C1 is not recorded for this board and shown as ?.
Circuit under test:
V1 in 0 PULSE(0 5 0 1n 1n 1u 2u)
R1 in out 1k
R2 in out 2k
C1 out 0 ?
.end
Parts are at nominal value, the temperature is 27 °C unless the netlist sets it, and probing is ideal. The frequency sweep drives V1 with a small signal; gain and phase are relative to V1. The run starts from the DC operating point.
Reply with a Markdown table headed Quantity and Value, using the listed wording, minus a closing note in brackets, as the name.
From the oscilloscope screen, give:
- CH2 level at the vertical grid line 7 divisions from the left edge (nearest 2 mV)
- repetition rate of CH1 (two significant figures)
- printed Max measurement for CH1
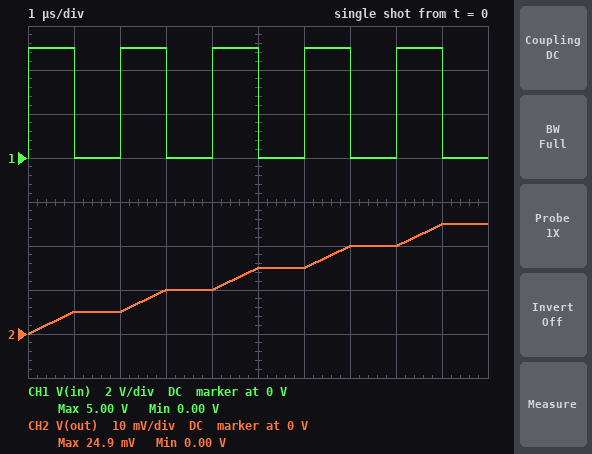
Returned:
| Quantity | Value |
|---|---|
| CH2 level at the vertical grid line 7 divisions from the left edge | 20 mV |
| repetition rate of CH1 | 500 kHz |
| printed Max measurement for CH1 | 5.00 V |
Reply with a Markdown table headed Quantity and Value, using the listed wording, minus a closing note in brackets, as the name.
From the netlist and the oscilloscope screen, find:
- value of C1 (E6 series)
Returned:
| Quantity | Value |
|---|---|
| value of C1 | 1.5 µF |
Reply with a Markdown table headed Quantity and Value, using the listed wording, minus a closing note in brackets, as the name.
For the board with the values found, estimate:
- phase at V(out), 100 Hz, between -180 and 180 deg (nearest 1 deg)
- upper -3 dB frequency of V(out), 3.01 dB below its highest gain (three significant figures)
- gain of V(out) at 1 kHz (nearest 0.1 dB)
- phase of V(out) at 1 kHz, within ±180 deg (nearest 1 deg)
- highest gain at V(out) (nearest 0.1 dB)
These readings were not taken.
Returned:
| Quantity | Value |
|---|---|
| phase at V(out), 100 Hz, between -180 and 180 deg | -32 deg |
| upper -3 dB frequency of V(out), 3.01 dB below its highest gain | 159 Hz |
| gain of V(out) at 1 kHz | -16.1 dB |
| phase of V(out) at 1 kHz, within ±180 deg | -81 deg |
| highest gain at V(out) | 0 dB |
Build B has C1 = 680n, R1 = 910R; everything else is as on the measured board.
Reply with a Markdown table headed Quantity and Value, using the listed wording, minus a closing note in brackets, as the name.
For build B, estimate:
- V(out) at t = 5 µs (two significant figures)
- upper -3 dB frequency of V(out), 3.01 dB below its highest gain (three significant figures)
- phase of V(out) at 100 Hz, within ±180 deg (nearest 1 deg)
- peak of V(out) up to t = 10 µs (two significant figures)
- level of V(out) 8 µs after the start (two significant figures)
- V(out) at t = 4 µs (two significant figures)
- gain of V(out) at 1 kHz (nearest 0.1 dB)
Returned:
| Quantity | Value |
|---|---|
| V(out) at t = 5 µs | 35 mV |
| upper -3 dB frequency of V(out), 3.01 dB below its highest gain | 374 Hz |
| phase of V(out) at 100 Hz, within ±180 deg | -15 deg |
| peak of V(out) up to t = 10 µs | 58 mV |
| level of V(out) 8 µs after the start | 47 mV |
| V(out) at t = 4 µs | 23 mV |
| gain of V(out) at 1 kHz | -9.1 dB |
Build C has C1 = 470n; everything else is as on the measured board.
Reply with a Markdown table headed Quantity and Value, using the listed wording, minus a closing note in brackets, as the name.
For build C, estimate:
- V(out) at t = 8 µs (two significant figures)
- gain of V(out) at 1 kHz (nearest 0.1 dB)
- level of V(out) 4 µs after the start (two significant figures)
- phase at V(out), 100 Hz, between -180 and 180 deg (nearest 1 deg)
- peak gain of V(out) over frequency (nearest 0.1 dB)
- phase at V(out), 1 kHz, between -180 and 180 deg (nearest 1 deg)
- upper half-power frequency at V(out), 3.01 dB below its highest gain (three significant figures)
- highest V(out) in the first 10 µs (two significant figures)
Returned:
| Quantity | Value |
|---|---|
| V(out) at t = 8 µs | 63 mV |
| gain of V(out) at 1 kHz | -6.9 dB |
| level of V(out) 4 µs after the start | 32 mV |
| phase at V(out), 100 Hz, between -180 and 180 deg | -11 deg |
| peak gain of V(out) over frequency | 0 dB |
| phase at V(out), 1 kHz, between -180 and 180 deg | -63 deg |
| upper half-power frequency at V(out), 3.01 dB below its highest gain | 508 Hz |
| highest V(out) in the first 10 µs | 79 mV |
